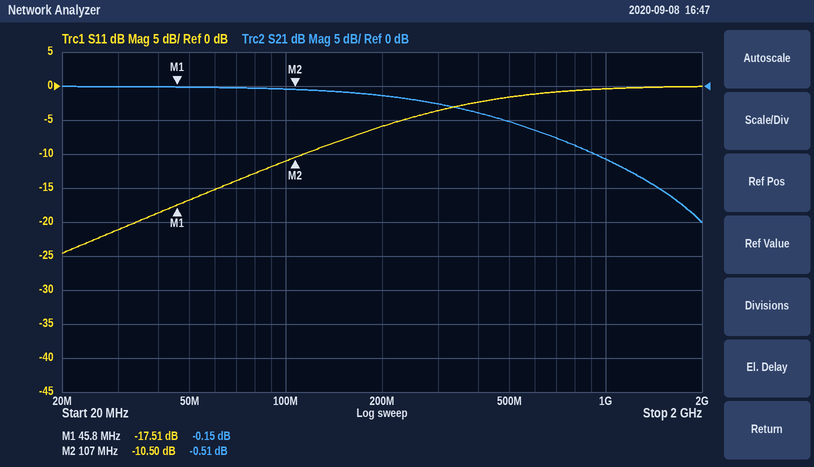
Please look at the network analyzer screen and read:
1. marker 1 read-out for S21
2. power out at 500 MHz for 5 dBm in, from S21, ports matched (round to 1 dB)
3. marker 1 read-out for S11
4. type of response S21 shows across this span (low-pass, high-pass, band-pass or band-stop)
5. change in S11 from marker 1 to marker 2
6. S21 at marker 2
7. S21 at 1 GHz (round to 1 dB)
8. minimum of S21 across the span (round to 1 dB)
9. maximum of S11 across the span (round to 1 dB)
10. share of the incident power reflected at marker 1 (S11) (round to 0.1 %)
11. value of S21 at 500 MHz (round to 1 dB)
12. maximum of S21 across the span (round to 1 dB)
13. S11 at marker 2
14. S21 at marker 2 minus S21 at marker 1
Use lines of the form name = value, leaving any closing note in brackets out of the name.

marker 1 read-out for S21 = -0.15 dB
power out at 500 MHz for 5 dBm in, from S21, ports matched = 0 dBm
marker 1 read-out for S11 = -17.51 dB
type of response S21 shows across this span = low-pass
change in S11 from marker 1 to marker 2 = 7.01 dB
S21 at marker 2 = -0.51 dB
S21 at 1 GHz = -11 dB
minimum of S21 across the span = -20 dB
maximum of S11 across the span = 0 dB
share of the incident power reflected at marker 1 (S11) = 1.8 %
value of S21 at 500 MHz = -5 dB
maximum of S21 across the span = 0 dB
S11 at marker 2 = -10.50 dB
S21 at marker 2 minus S21 at marker 1 = -0.36 dB
